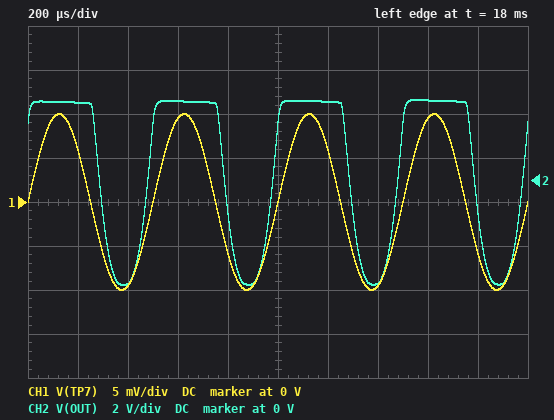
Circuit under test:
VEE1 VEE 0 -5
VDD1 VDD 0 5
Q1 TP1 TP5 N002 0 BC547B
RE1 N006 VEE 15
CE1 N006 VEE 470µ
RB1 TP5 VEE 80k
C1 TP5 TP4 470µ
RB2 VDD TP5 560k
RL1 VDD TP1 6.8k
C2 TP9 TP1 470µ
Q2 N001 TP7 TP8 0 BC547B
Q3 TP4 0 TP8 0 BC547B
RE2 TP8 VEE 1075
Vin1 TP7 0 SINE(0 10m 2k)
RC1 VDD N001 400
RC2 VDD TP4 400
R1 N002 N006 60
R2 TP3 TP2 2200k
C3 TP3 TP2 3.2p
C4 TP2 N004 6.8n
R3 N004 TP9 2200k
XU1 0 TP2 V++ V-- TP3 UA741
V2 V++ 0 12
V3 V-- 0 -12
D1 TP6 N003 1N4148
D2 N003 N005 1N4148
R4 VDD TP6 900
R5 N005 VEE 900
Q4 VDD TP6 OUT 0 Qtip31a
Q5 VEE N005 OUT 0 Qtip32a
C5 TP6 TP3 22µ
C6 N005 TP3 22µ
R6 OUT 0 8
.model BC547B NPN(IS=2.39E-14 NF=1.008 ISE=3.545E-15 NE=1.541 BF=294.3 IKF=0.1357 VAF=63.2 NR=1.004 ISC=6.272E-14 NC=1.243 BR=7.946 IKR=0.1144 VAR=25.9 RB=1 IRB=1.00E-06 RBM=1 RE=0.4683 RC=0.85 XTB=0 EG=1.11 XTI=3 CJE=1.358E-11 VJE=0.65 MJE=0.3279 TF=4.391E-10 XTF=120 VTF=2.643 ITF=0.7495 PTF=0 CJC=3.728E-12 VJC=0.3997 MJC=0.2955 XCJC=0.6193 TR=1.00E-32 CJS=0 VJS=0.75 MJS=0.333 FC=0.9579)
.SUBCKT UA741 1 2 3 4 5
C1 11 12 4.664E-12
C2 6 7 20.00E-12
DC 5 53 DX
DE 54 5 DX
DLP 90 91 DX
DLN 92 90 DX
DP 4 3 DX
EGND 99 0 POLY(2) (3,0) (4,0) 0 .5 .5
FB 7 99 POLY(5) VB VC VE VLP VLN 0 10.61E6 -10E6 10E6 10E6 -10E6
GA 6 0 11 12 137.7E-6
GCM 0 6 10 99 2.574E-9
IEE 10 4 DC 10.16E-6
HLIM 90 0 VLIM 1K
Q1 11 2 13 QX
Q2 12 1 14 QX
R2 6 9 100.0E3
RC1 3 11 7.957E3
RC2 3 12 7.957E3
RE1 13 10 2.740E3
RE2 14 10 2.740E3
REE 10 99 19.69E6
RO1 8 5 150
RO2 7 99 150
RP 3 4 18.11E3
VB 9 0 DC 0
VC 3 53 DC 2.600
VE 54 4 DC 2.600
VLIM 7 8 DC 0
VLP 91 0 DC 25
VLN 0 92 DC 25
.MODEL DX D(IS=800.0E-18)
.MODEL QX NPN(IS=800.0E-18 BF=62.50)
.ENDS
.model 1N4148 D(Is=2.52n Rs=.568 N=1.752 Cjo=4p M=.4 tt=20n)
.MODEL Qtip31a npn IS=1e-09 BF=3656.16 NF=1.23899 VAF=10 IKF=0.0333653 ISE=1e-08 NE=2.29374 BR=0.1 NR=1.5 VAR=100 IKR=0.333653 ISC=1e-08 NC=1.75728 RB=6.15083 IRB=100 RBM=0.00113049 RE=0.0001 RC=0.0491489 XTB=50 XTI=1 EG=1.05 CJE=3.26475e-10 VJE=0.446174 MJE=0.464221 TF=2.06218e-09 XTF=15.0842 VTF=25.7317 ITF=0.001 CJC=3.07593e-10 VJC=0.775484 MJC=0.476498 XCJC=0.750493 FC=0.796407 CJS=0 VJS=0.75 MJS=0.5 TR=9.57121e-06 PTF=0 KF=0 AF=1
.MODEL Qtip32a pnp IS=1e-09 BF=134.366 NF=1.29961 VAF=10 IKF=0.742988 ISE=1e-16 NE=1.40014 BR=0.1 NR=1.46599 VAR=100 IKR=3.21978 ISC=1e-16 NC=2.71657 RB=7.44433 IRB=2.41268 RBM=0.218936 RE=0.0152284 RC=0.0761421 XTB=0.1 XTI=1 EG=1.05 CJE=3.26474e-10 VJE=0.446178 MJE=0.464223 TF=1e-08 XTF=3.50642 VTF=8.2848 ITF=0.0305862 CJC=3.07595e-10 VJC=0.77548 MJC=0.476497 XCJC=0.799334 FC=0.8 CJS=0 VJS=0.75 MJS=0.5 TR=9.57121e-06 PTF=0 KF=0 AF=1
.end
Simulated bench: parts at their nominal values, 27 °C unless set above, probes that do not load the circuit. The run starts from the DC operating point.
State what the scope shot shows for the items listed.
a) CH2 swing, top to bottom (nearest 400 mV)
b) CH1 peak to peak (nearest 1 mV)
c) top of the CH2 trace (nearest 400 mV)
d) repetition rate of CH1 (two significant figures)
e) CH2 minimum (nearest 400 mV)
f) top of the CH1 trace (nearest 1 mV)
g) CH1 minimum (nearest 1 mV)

8.4 V
20 mV
3.6 V
2.0 kHz
-4.8 V
10 mV
-10 mV
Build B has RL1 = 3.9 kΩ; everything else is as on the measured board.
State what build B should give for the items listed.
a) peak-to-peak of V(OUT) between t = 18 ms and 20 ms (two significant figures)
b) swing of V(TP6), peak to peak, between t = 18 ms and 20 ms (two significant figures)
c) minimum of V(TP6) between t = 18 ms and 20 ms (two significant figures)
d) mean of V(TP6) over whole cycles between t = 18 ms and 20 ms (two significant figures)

8.2 V
8.4 V
-4.0 V
1.0 V
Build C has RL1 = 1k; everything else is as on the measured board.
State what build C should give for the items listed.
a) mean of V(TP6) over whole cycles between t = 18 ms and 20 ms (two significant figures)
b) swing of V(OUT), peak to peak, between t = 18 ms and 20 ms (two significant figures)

770 mV
3.5 V
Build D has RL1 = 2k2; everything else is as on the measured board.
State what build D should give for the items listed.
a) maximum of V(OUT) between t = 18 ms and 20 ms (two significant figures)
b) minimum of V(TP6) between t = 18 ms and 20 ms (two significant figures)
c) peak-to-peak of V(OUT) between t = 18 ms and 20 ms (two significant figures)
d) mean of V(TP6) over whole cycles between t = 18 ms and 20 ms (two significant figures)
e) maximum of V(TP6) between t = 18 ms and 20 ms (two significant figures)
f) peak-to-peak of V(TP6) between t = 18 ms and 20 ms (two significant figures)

4.1 V
-2.9 V
7.5 V
760 mV
4.8 V
7.7 V
